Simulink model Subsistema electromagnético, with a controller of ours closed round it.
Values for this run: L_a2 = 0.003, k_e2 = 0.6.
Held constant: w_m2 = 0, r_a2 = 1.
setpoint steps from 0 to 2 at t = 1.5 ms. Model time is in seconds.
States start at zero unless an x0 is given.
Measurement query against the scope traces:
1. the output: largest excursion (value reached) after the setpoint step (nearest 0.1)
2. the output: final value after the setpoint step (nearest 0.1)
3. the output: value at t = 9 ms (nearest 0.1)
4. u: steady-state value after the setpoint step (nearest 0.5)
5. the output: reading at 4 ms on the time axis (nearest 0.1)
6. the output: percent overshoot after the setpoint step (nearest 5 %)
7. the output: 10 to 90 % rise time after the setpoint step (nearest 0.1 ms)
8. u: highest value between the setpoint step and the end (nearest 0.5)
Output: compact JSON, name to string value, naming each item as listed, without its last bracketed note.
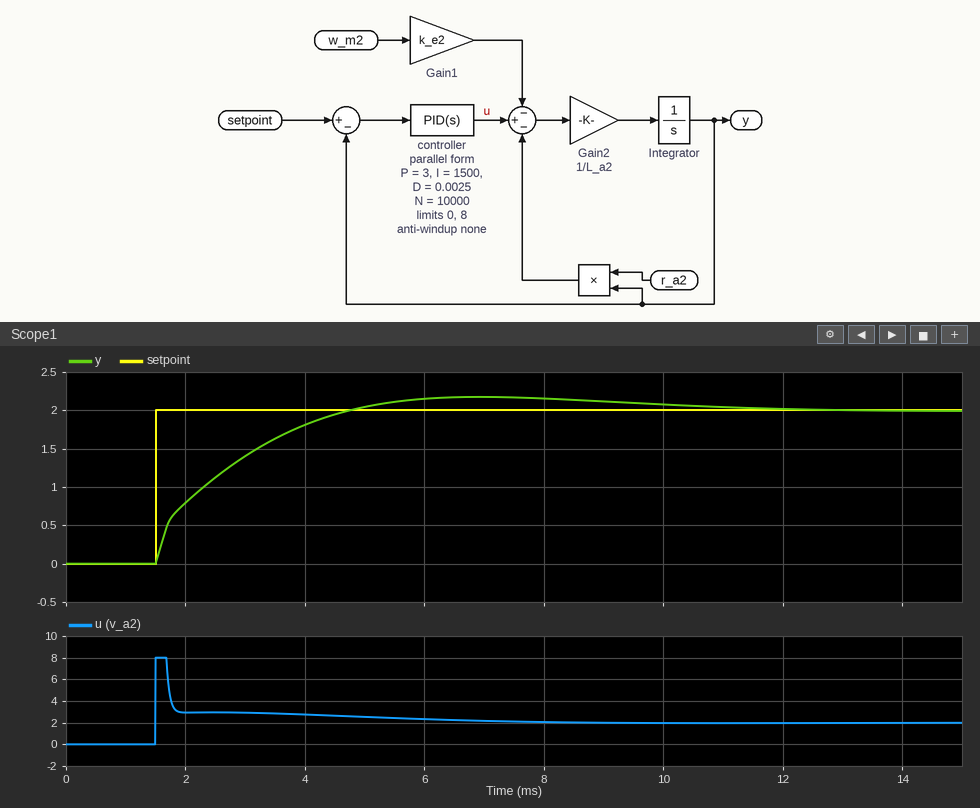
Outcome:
{"the output: largest excursion (value reached) after the setpoint step": "2.2", "the output: final value after the setpoint step": "2.0", "the output: value at t = 9 ms": "2.1", "u: steady-state value after the setpoint step": "2.0", "the output: reading at 4 ms on the time axis": "1.8", "the output: percent overshoot after the setpoint step": "10 %", "the output: 10 to 90 % rise time after the setpoint step": "2.4 ms", "u: highest value between the setpoint step and the end": "8.0"}
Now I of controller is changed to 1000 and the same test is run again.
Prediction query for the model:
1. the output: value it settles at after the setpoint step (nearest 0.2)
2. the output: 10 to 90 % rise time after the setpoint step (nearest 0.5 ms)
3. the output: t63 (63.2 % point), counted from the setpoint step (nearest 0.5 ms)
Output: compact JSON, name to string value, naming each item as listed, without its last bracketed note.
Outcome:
{"the output: value it settles at after the setpoint step": "2.0", "the output: 10 to 90 % rise time after the setpoint step": "3.0 ms", "the output: t63 (63.2 % point), counted from the setpoint step": "1.5 ms"}
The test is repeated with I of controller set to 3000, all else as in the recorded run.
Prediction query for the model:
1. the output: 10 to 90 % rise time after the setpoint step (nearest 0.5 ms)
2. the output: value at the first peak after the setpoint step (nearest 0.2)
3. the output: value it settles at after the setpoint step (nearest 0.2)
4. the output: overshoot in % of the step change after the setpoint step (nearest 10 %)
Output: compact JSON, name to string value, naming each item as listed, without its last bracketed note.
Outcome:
{"the output: 10 to 90 % rise time after the setpoint step": "1.5 ms", "the output: value at the first peak after the setpoint step": "2.4", "the output: value it settles at after the setpoint step": "2.0", "the output: overshoot in % of the step change after the setpoint step": "20 %"}
